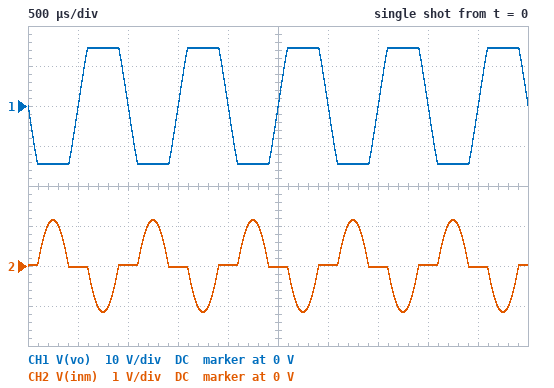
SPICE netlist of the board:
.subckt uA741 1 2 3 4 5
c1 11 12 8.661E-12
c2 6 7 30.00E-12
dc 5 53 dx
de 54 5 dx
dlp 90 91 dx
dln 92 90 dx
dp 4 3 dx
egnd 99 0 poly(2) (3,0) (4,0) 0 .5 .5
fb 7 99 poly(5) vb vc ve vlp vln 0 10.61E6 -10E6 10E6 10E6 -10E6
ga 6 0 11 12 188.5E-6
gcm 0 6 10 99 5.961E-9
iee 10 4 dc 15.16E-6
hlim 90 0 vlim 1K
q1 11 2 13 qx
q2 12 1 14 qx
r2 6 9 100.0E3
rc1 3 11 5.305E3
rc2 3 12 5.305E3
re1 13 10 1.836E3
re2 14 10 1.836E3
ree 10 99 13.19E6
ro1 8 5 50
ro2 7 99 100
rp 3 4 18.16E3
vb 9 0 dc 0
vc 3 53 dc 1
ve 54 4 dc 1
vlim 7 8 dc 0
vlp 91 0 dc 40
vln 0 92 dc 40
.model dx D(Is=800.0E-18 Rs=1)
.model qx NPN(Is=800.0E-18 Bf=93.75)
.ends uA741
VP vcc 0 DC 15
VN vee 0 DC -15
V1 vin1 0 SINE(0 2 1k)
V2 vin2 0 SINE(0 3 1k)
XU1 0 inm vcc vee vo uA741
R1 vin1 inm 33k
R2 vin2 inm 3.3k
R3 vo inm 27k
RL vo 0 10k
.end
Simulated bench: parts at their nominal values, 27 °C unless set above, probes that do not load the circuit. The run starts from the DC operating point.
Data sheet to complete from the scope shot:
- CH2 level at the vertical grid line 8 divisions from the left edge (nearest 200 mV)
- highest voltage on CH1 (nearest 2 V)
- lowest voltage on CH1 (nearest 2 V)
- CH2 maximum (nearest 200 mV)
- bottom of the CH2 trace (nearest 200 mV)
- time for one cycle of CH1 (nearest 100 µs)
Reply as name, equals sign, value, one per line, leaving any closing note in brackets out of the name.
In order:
CH2 level at the vertical grid line 8 divisions from the left edge = 0 V
highest voltage on CH1 = 14 V
lowest voltage on CH1 = -14 V
CH2 maximum = 1.2 V
bottom of the CH2 trace = -1.2 V
time for one cycle of CH1 = 1.0 ms
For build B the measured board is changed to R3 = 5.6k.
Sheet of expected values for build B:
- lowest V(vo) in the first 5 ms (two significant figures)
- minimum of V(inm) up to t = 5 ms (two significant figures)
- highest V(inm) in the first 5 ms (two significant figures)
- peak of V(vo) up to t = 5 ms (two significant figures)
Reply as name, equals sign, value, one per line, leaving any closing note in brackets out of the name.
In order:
lowest V(vo) in the first 5 ms = -5.4 V
minimum of V(inm) up to t = 5 ms = -5.5 mV
highest V(inm) in the first 5 ms = 5.5 mV
peak of V(vo) up to t = 5 ms = 5.4 V
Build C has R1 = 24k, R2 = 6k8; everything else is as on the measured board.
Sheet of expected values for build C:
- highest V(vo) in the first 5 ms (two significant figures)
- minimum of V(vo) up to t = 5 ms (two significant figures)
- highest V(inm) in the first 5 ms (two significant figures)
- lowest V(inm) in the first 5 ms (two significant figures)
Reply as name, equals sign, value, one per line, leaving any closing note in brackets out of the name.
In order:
highest V(vo) in the first 5 ms = 14 V
minimum of V(vo) up to t = 5 ms = -14 V
highest V(inm) in the first 5 ms = 14 mV
lowest V(inm) in the first 5 ms = -14 mV
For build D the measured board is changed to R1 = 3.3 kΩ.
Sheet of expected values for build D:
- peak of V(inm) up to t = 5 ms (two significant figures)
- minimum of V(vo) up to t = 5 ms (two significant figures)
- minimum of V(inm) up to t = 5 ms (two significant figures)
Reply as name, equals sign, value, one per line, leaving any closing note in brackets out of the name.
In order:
peak of V(inm) up to t = 5 ms = 1.5 V
minimum of V(vo) up to t = 5 ms = -15 V
minimum of V(inm) up to t = 5 ms = -1.5 V
